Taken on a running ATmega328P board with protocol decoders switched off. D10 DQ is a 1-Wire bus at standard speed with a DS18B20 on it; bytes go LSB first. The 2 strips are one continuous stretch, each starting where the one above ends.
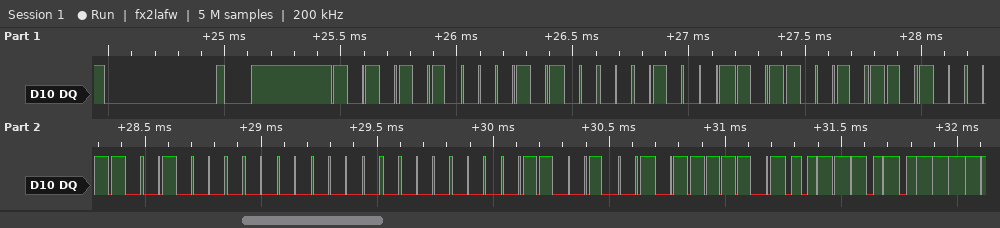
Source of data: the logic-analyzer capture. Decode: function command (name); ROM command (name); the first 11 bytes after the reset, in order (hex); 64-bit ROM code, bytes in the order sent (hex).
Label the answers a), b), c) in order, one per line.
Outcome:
a) Read Scratchpad
b) Match ROM
c) 55 28 88 4D 8B 09 00 00 93 BE 5C
d) 28 88 4D 8B 09 00 00 93
